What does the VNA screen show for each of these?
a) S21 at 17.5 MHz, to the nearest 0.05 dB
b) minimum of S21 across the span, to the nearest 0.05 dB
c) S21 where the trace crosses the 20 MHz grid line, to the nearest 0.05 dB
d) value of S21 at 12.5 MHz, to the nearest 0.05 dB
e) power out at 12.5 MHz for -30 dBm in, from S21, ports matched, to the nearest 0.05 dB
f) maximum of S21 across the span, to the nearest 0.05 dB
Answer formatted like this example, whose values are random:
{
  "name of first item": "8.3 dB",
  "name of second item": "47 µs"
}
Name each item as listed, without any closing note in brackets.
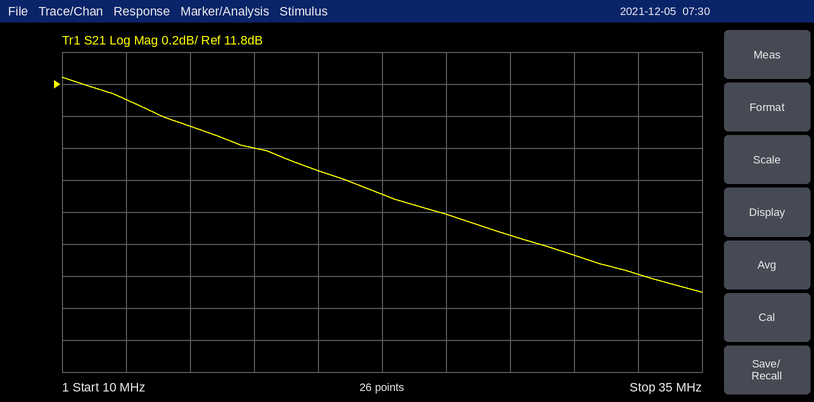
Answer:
{
  "S21 at 17.5 MHz, to the nearest 0.05 dB": "11.40 dB",
  "minimum of S21 across the span, to the nearest 0.05 dB": "10.50 dB",
  "S21 where the trace crosses the 20 MHz grid line, to the nearest 0.05 dB": "11.25 dB",
  "value of S21 at 12.5 MHz, to the nearest 0.05 dB": "11.70 dB",
  "power out at 12.5 MHz for -30 dBm in, from S21, ports matched, to the nearest 0.05 dB": "-18.30 dBm",
  "maximum of S21 across the span, to the nearest 0.05 dB": "11.85 dB"
}
